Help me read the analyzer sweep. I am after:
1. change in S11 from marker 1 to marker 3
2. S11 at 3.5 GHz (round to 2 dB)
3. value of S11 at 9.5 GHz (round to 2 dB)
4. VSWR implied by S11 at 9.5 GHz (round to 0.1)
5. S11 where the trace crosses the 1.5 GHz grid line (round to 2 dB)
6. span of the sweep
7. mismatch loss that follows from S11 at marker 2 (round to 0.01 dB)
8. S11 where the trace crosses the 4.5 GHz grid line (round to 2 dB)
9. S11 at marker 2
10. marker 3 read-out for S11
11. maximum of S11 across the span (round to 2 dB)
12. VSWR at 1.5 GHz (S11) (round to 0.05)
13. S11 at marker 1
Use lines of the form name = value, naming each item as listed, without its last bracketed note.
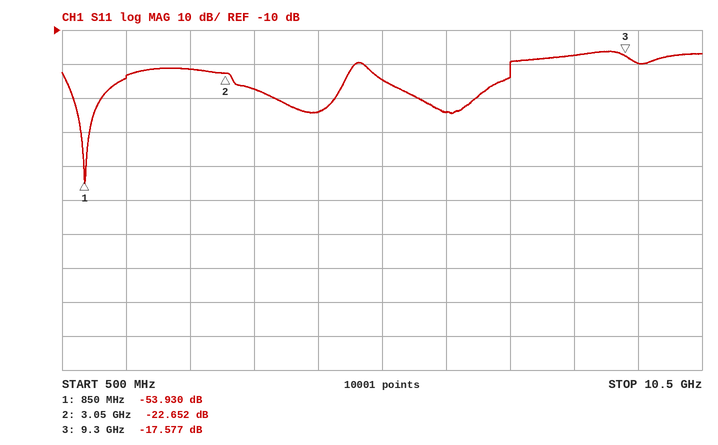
change in S11 from marker 1 to marker 3 = 36.353 dB
S11 at 3.5 GHz = -28 dB
value of S11 at 9.5 GHz = -20 dB
VSWR implied by S11 at 9.5 GHz = 1.2
S11 where the trace crosses the 1.5 GHz grid line = -24 dB
span of the sweep = 10 GHz
mismatch loss that follows from S11 at marker 2 = 0.02 dB
S11 where the trace crosses the 4.5 GHz grid line = -34 dB
S11 at marker 2 = -22.652 dB
marker 3 read-out for S11 = -17.577 dB
maximum of S11 across the span = -16 dB
VSWR at 1.5 GHz (S11) = 1.15
S11 at marker 1 = -53.930 dB
